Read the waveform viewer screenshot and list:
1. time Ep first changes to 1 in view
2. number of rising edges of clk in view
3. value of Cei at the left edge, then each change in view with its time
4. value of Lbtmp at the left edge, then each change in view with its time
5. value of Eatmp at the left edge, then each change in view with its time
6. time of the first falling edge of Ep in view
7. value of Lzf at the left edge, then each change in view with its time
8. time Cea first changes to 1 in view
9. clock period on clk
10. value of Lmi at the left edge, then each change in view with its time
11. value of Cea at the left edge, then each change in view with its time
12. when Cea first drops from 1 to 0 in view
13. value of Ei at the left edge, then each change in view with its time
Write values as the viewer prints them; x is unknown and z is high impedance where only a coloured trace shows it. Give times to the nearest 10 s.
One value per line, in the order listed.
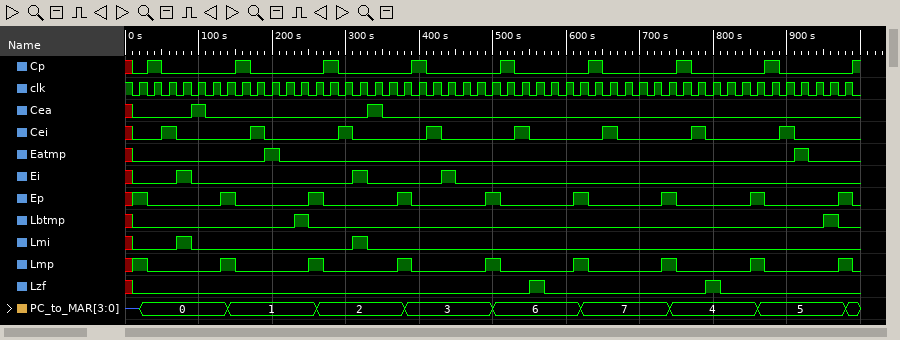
10 s
49
x, 0 at 10 s, 1 at 50 s, 0 at 70 s, 1 at 170 s, 0 at 190 s, 1 at 290 s, 0 at 310 s, 1 at 410 s, 0 at 430 s, 1 at 530 s, 0 at 550 s, 1 at 650 s, 0 at 670 s, 1 at 770 s, 0 at 790 s, 1 at 890 s, 0 at 910 s
x, 0 at 10 s, 1 at 230 s, 0 at 250 s, 1 at 950 s, 0 at 970 s
x, 0 at 10 s, 1 at 190 s, 0 at 210 s, 1 at 910 s, 0 at 930 s
30 s
x, 0 at 10 s, 1 at 550 s, 0 at 570 s, 1 at 790 s, 0 at 810 s
90 s
20 s
x, 0 at 10 s, 1 at 70 s, 0 at 90 s, 1 at 310 s, 0 at 330 s
x, 0 at 10 s, 1 at 90 s, 0 at 110 s, 1 at 330 s, 0 at 350 s
110 s
x, 0 at 10 s, 1 at 70 s, 0 at 90 s, 1 at 310 s, 0 at 330 s, 1 at 430 s, 0 at 450 s
